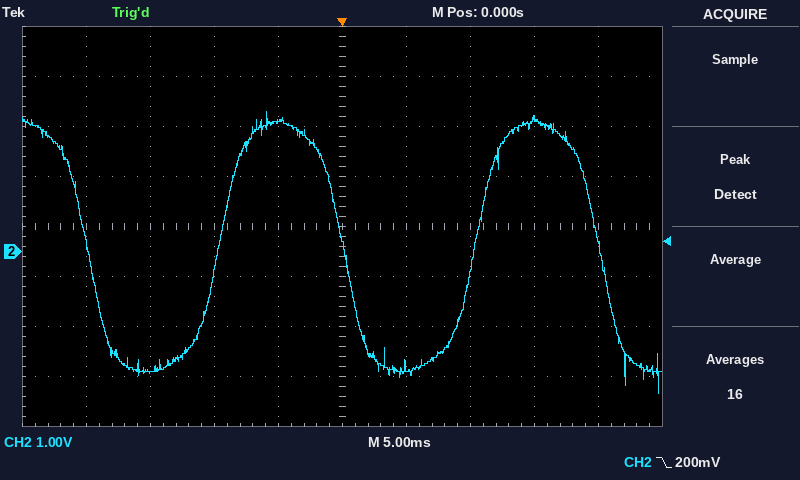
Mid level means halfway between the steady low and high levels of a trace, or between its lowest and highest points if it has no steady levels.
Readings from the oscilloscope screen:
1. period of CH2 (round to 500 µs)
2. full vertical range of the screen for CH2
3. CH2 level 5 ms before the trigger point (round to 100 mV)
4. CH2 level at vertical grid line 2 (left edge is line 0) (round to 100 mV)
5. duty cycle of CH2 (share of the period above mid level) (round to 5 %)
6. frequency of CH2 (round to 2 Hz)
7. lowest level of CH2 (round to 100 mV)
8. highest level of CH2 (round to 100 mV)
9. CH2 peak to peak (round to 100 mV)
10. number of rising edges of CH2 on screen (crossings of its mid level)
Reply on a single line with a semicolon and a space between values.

20.0 ms; 8 V; 2.6 V; -2.4 V; 50 %; 50 Hz; -2.8 V; 2.8 V; 5.6 V; 2
